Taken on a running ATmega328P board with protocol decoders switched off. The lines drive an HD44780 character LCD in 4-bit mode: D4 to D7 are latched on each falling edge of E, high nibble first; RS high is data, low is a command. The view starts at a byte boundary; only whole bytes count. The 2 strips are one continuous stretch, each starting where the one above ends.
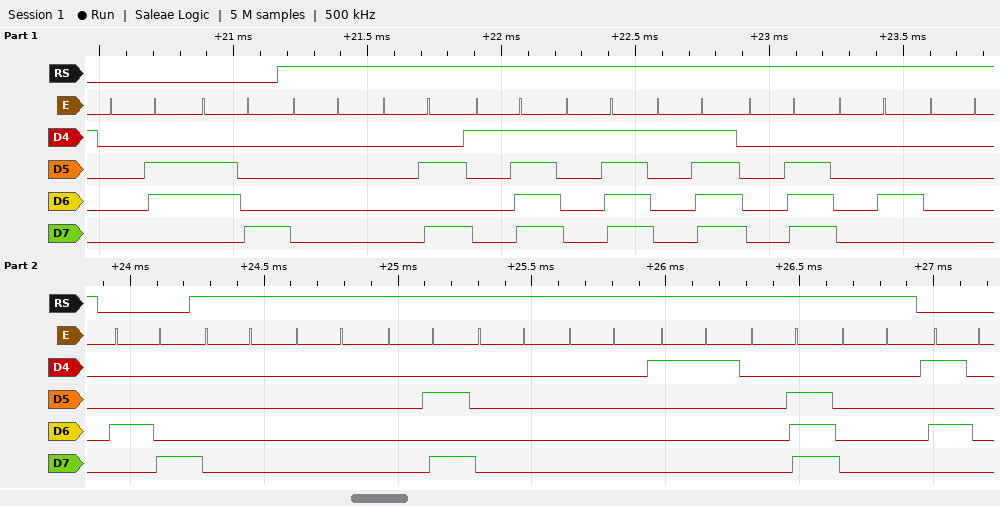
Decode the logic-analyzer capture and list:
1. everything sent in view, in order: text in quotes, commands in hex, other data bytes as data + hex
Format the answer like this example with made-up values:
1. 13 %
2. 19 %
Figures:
1. 0x06 0x68 data 00 0A 1F 1F 1F 0E 04 00 0x48 data 00 00 0A 00 00 11 0E 00 0x50
